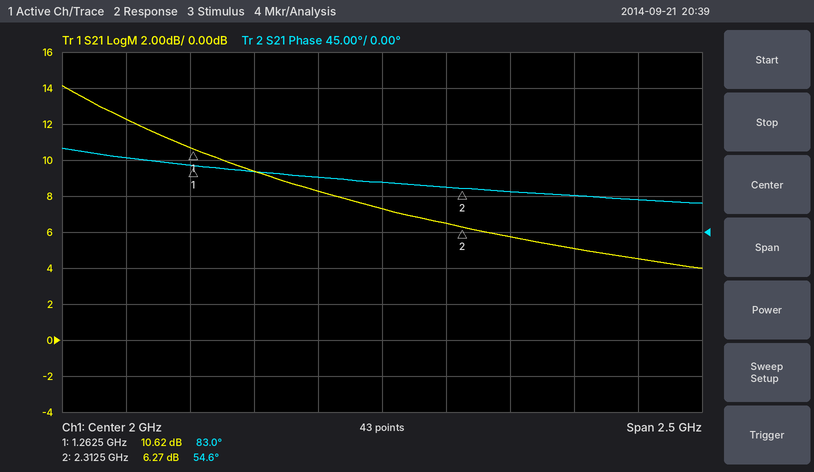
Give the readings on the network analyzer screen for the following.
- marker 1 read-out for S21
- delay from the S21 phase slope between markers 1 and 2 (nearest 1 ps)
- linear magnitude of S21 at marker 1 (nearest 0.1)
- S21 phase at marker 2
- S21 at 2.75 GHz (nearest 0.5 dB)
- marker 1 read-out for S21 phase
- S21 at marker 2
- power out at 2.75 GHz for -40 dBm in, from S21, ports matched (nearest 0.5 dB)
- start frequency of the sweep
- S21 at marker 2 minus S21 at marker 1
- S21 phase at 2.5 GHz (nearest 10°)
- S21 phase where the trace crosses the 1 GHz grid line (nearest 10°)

10.62 dB
75 ps
3.4
54.6°
5.0 dB
83.0°
6.27 dB
-35.0 dBm
750 MHz
-4.35 dB
50°
90°
